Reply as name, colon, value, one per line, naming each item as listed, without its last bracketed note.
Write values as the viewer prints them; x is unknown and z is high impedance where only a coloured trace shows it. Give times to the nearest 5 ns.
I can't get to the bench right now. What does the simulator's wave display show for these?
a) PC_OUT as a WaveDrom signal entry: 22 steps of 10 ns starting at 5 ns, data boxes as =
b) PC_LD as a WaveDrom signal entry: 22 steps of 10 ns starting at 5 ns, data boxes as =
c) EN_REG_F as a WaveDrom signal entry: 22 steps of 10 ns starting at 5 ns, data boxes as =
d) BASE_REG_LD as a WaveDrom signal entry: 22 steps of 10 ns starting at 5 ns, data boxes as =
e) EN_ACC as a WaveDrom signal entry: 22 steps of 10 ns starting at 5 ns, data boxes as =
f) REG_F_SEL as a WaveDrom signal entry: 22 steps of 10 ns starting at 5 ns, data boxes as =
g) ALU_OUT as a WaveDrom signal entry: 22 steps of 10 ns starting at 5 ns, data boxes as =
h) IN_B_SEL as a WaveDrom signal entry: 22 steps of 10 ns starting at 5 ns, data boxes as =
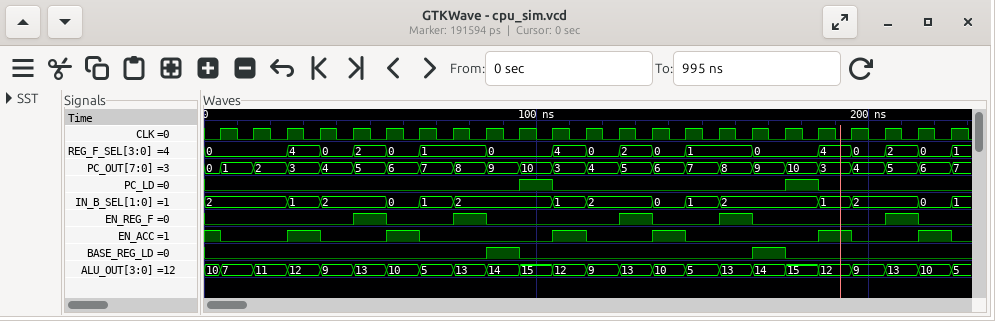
PC_OUT as a WaveDrom signal entry: 22 steps of 10 ns starting at 5 ns, data boxes as =: {name: 'PC_OUT', wave: '======================', data: '1 2 3 4 5 6 7 8 9 10 3 4 5 6 7 8 9 10 3 4 5 6'}
PC_LD as a WaveDrom signal entry: 22 steps of 10 ns starting at 5 ns, data boxes as =: {name: 'PC_LD', wave: '0........10......10...'}
EN_REG_F as a WaveDrom signal entry: 22 steps of 10 ns starting at 5 ns, data boxes as =: {name: 'EN_REG_F', wave: '0...10.10...10.10...10'}
BASE_REG_LD as a WaveDrom signal entry: 22 steps of 10 ns starting at 5 ns, data boxes as =: {name: 'BASE_REG_LD', wave: '0.......10......10....'}
EN_ACC as a WaveDrom signal entry: 22 steps of 10 ns starting at 5 ns, data boxes as =: {name: 'EN_ACC', wave: '0.10.10...10.10...10.1'}
REG_F_SEL as a WaveDrom signal entry: 22 steps of 10 ns starting at 5 ns, data boxes as =: {name: 'REG_F_SEL', wave: '=.=====.=.=====.=.====', data: '0 4 0 2 0 1 0 4 0 2 0 1 0 4 0 2 0'}
ALU_OUT as a WaveDrom signal entry: 22 steps of 10 ns starting at 5 ns, data boxes as =: {name: 'ALU_OUT', wave: '======================', data: '7 11 12 9 13 10 5 13 14 15 12 9 13 10 5 13 14 15 12 9 13 10'}
IN_B_SEL as a WaveDrom signal entry: 22 steps of 10 ns starting at 5 ns, data boxes as =: {name: 'IN_B_SEL', wave: '=.==.===..==.===..==.=', data: '2 1 2 0 1 2 1 2 0 1 2 1 2 0'}
